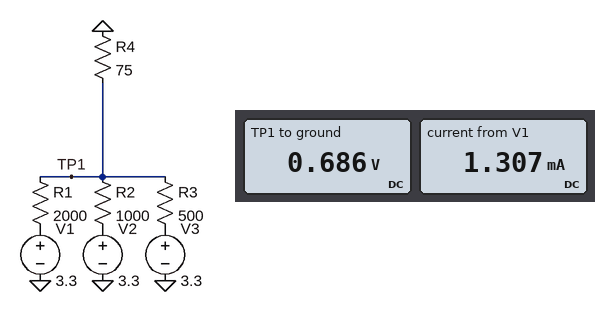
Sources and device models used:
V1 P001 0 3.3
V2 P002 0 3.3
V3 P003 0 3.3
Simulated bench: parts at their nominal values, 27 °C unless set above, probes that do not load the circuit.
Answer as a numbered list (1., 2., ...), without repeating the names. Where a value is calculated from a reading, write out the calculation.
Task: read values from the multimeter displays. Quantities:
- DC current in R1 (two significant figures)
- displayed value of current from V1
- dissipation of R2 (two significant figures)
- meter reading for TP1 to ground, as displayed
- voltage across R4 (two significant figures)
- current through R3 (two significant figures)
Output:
1. (3.3 V - 686 mV) / 2 kΩ = 1.3 mA
2. 1.307 mA
3. (3.3 V - 686 mV)^2 / 1 kΩ = 6.8 mW
4. 0.686 V
5. 686 mV = 690 mV
6. (3.3 V - 686 mV) / 500 Ω = 5.2 mA
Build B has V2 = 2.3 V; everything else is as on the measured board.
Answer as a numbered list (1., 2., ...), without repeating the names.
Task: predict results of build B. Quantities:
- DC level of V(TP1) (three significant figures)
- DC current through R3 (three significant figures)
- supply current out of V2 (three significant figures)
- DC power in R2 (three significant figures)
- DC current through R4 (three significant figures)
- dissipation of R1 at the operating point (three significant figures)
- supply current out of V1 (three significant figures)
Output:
1. 627 mV
2. 5.35 mA
3. 1.67 mA
4. 2.80 mW
5. 8.36 mA
6. 3.57 mW
7. 1.34 mA
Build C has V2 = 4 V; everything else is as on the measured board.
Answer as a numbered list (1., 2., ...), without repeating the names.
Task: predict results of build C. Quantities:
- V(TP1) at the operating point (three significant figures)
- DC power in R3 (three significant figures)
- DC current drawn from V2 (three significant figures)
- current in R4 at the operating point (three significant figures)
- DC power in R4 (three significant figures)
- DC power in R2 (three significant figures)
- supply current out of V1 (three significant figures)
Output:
1. 728 mV
2. 13.2 mW
3. 3.27 mA
4. 9.70 mA
5. 7.06 mW
6. 10.7 mW
7. 1.29 mA
